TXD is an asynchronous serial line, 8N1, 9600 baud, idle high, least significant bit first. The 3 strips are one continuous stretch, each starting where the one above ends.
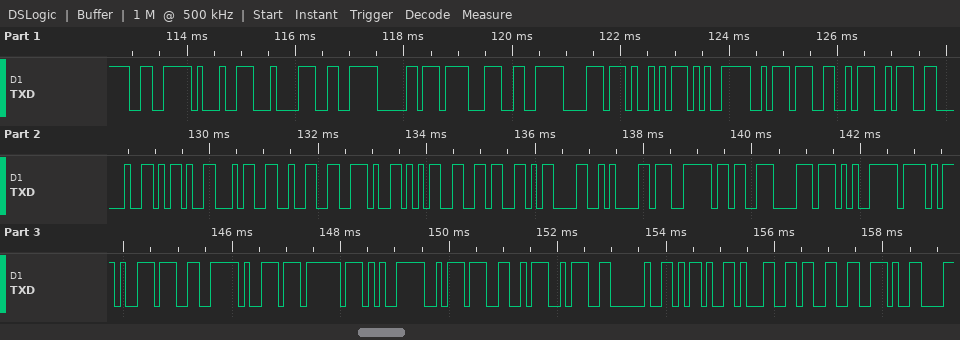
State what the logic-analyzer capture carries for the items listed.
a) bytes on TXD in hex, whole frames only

E6 91 84 E6 B0 8F E6 B8 A9 E5 BA A6 3A 20 2D 34 32 2E 35 36 0D 0A E7 9B B8 E5 AF B9 E6 B9 BF E5 BA A6 3A 20 2D 31 33 2E
